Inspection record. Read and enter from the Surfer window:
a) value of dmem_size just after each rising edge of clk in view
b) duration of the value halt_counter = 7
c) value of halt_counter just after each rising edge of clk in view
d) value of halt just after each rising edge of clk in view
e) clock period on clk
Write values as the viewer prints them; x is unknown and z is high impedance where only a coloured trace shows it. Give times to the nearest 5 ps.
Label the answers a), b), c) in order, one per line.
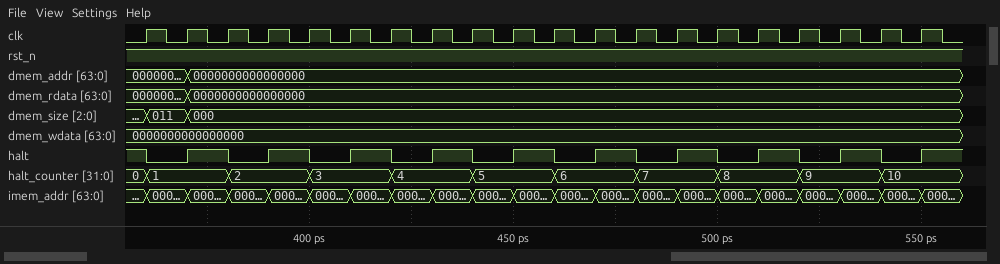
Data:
a) 011, 000, 000, 000, 000, 000, 000, 000, 000, 000, 000, 000, 000, 000, 000, 000, 000, 000, 000, 000
b) 20 ps
c) 1, 1, 2, 2, 3, 3, 4, 4, 5, 5, 6, 6, 7, 7, 8, 8, 9, 9, 10, 10
d) 0 1 0 1 0 1 0 1 0 1 0 1 0 1 0 1 0 1 0 1
e) 10 ps
